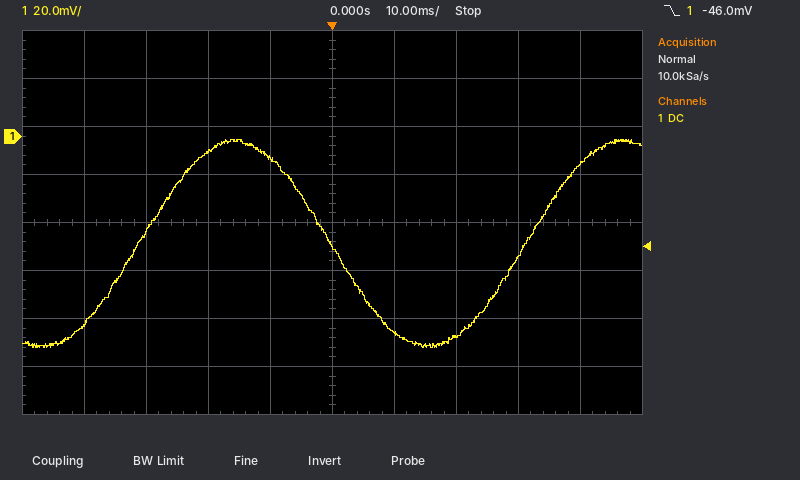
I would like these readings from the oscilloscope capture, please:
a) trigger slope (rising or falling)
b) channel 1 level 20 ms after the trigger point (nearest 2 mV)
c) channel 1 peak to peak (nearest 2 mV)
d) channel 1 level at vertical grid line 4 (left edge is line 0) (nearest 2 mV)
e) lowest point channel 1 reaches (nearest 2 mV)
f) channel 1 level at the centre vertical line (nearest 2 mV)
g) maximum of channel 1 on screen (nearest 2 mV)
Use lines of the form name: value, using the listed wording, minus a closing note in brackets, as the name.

trigger slope: falling
channel 1 level 20 ms after the trigger point: -84 mV
channel 1 peak to peak: 86 mV
channel 1 level at vertical grid line 4 (left edge is line 0): -10 mV
lowest point channel 1 reaches: -88 mV
channel 1 level at the centre vertical line: -46 mV
maximum of channel 1 on screen: -2 mV
